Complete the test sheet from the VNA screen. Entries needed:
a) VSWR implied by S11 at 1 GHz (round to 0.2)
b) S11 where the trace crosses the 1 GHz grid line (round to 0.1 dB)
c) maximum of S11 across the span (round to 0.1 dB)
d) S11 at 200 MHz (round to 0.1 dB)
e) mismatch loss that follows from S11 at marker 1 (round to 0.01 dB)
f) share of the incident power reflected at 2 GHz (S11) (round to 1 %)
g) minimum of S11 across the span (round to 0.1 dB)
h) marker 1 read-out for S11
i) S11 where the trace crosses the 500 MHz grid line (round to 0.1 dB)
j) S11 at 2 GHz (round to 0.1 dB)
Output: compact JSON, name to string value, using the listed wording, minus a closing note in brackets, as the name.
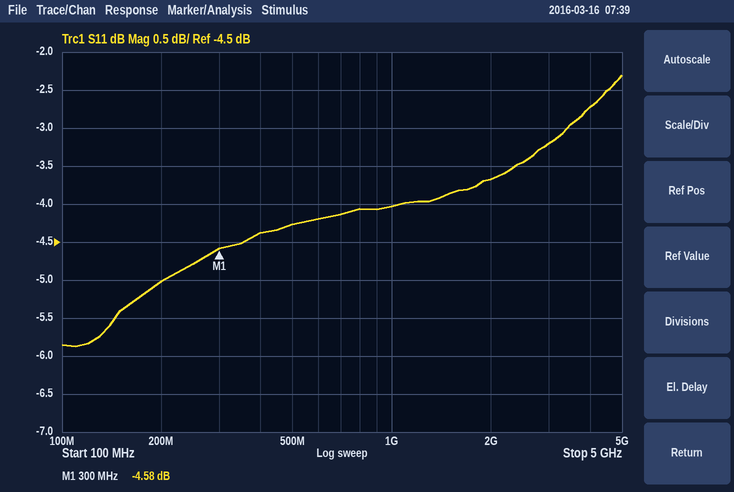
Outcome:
{"VSWR implied by S11 at 1 GHz": "4.4", "S11 where the trace crosses the 1 GHz grid line": "-4.0 dB", "maximum of S11 across the span": "-2.3 dB", "S11 at 200 MHz": "-5.0 dB", "mismatch loss that follows from S11 at marker 1": "1.86 dB", "share of the incident power reflected at 2 GHz (S11)": "43 %", "minimum of S11 across the span": "-5.9 dB", "marker 1 read-out for S11": "-4.58 dB", "S11 where the trace crosses the 500 MHz grid line": "-4.3 dB", "S11 at 2 GHz": "-3.7 dB"}
